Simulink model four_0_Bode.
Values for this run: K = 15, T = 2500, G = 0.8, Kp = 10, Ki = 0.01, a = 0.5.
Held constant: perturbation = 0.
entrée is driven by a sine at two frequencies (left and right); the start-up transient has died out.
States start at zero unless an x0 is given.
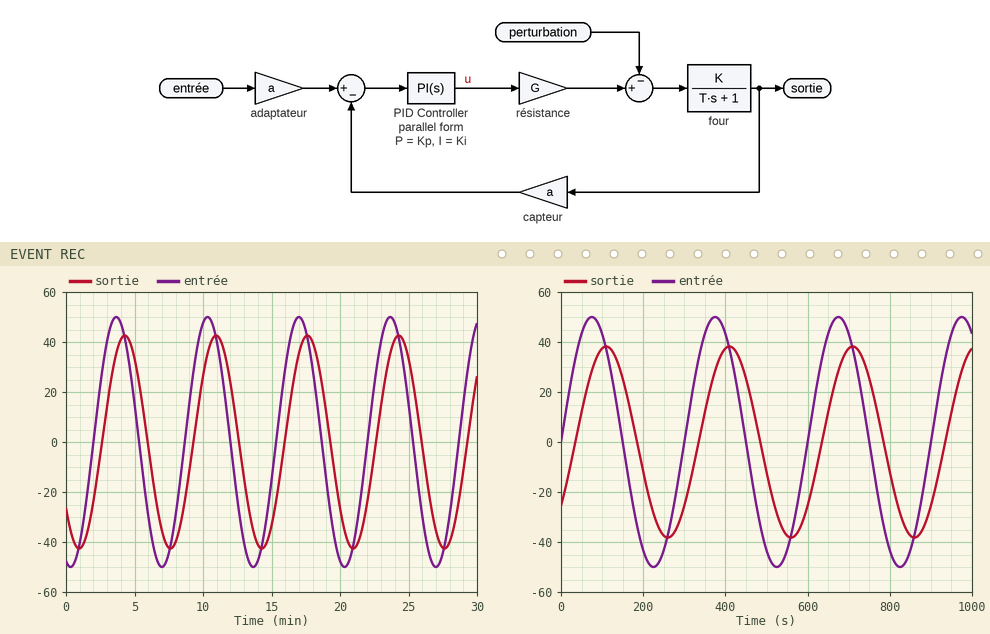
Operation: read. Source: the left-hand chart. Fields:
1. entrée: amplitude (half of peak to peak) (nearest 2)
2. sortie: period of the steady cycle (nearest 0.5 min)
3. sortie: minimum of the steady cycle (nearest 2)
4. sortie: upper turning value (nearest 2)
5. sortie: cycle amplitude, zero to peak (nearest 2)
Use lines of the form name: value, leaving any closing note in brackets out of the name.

entrée: amplitude (half of peak to peak): 50
sortie: period of the steady cycle: 6.5 min
sortie: minimum of the steady cycle: -42
sortie: upper turning value: 42
sortie: cycle amplitude, zero to peak: 42
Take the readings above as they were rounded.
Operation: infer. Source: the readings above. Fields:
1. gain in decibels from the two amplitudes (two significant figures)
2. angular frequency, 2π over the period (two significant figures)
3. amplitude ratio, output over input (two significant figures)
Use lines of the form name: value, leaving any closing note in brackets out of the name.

gain in decibels from the two amplitudes: -1.5 dB
angular frequency, 2π over the period: 0.97 rad/min
amplitude ratio, output over input: 0.84
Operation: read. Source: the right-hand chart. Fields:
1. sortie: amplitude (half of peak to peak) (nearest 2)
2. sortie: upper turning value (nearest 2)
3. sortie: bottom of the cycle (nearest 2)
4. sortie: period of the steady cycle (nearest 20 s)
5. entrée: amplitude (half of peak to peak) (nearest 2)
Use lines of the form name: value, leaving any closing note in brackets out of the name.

sortie: amplitude (half of peak to peak): 38
sortie: upper turning value: 38
sortie: bottom of the cycle: -38
sortie: period of the steady cycle: 300 s
entrée: amplitude (half of peak to peak): 50
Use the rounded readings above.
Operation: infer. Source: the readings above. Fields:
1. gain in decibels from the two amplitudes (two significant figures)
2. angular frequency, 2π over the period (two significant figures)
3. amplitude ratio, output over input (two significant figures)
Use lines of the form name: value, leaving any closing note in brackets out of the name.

gain in decibels from the two amplitudes: -2.4 dB
angular frequency, 2π over the period: 0.021 rad/s
amplitude ratio, output over input: 0.76
